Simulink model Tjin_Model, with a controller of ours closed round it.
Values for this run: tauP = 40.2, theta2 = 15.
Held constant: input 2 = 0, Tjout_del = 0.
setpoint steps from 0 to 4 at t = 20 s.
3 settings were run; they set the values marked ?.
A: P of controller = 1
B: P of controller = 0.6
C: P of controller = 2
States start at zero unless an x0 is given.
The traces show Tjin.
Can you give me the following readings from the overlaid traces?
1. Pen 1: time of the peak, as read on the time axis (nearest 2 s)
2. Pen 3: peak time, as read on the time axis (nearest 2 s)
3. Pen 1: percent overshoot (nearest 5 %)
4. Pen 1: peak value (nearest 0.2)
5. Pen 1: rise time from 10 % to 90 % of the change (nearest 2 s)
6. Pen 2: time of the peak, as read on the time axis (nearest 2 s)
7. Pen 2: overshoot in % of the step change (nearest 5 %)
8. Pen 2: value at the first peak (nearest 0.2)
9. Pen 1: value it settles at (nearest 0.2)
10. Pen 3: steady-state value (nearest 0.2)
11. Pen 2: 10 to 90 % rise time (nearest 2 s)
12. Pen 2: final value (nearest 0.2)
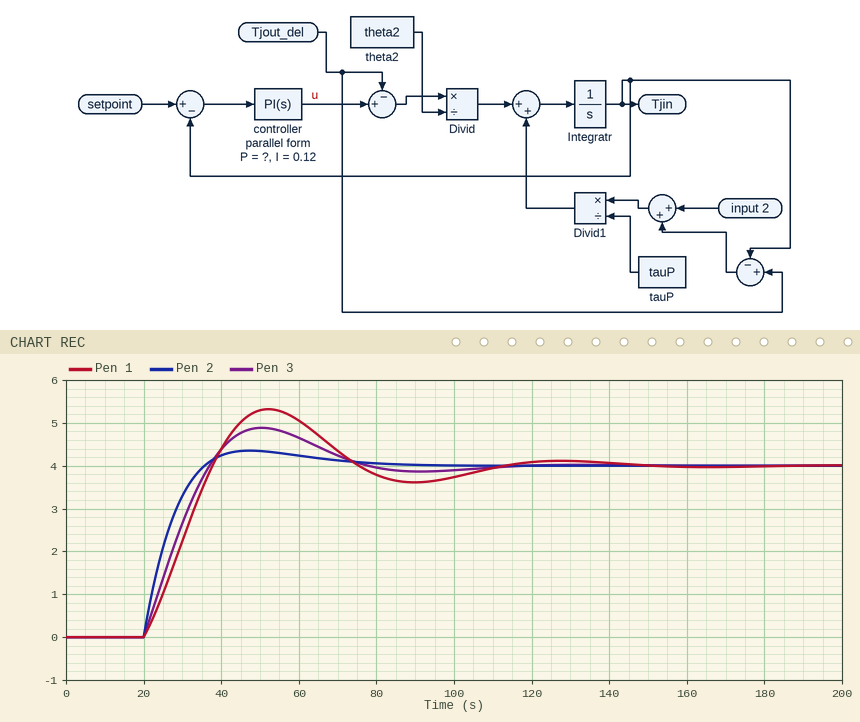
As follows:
52 s
50 s
35 %
5.4
14 s
48 s
10 %
4.4
4.0
4.0
12 s
4.0
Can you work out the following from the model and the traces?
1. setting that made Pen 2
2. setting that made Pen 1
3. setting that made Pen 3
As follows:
C
B
A
